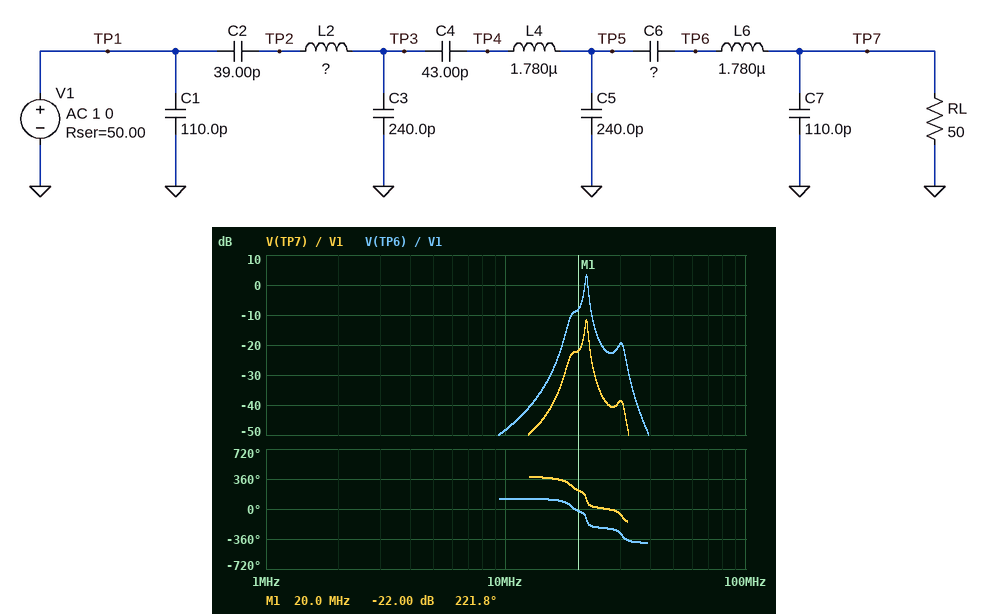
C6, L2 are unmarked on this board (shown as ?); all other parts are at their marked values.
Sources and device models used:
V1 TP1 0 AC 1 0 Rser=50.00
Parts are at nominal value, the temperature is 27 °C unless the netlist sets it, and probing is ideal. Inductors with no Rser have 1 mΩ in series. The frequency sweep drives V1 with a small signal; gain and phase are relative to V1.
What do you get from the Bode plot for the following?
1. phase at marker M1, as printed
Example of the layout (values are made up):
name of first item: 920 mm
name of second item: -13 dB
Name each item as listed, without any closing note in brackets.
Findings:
phase at marker M1, as printed: 221.8 deg
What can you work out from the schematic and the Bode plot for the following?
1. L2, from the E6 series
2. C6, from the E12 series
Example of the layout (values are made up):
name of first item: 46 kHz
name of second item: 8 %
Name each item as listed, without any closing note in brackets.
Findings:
L2, from the E6 series: 2.2 µH
C6, from the E12 series: 18 pF
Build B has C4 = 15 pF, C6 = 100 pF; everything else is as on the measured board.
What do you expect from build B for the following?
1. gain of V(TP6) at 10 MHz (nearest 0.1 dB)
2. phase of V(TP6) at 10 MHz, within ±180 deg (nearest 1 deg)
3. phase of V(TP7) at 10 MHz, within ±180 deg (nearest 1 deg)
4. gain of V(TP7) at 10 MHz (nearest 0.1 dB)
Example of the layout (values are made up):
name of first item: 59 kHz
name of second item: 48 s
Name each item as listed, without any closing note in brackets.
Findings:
gain of V(TP6) at 10 MHz: -41.1 dB
phase of V(TP6) at 10 MHz, within ±180 deg: 109 deg
phase of V(TP7) at 10 MHz, within ±180 deg: 25 deg
gain of V(TP7) at 10 MHz: -48.2 dB
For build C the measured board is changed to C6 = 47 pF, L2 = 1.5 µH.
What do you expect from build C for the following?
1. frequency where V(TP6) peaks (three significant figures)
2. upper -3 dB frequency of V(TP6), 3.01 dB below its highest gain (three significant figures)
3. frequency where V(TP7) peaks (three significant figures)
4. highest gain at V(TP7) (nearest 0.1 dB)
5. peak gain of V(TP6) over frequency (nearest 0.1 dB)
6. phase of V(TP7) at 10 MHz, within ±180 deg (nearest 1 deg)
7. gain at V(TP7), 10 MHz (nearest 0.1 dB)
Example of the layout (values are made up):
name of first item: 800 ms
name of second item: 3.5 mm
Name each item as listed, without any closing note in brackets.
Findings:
frequency where V(TP6) peaks: 21.5 MHz
upper -3 dB frequency of V(TP6), 3.01 dB below its highest gain: 22.5 MHz
frequency where V(TP7) peaks: 21.4 MHz
highest gain at V(TP7): -6.4 dB
peak gain of V(TP6) over frequency: 8.3 dB
phase of V(TP7) at 10 MHz, within ±180 deg: 37 deg
gain at V(TP7), 10 MHz: -47.3 dB
